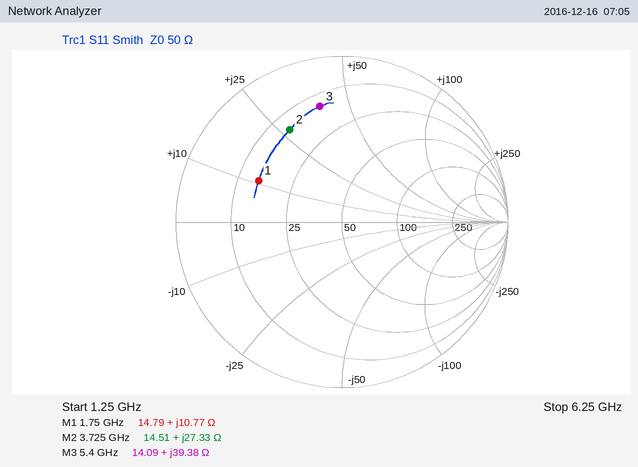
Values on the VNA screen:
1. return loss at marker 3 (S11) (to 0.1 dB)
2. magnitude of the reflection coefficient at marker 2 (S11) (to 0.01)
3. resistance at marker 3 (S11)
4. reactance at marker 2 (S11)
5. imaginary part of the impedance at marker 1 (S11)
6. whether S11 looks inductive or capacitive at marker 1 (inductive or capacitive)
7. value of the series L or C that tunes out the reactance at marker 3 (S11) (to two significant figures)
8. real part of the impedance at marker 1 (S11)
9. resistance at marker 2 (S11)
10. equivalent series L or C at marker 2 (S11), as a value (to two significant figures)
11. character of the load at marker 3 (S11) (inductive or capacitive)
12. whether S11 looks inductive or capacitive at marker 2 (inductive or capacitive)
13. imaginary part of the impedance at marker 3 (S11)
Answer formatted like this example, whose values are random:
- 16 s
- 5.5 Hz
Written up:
- 3.0 dB
- 0.64
- 14.09 Ω
- +27.33 Ω
- +10.77 Ω
- inductive
- 750 fF
- 14.79 Ω
- 14.51 Ω
- 1.2 nH
- inductive
- inductive
- +39.38 Ω
